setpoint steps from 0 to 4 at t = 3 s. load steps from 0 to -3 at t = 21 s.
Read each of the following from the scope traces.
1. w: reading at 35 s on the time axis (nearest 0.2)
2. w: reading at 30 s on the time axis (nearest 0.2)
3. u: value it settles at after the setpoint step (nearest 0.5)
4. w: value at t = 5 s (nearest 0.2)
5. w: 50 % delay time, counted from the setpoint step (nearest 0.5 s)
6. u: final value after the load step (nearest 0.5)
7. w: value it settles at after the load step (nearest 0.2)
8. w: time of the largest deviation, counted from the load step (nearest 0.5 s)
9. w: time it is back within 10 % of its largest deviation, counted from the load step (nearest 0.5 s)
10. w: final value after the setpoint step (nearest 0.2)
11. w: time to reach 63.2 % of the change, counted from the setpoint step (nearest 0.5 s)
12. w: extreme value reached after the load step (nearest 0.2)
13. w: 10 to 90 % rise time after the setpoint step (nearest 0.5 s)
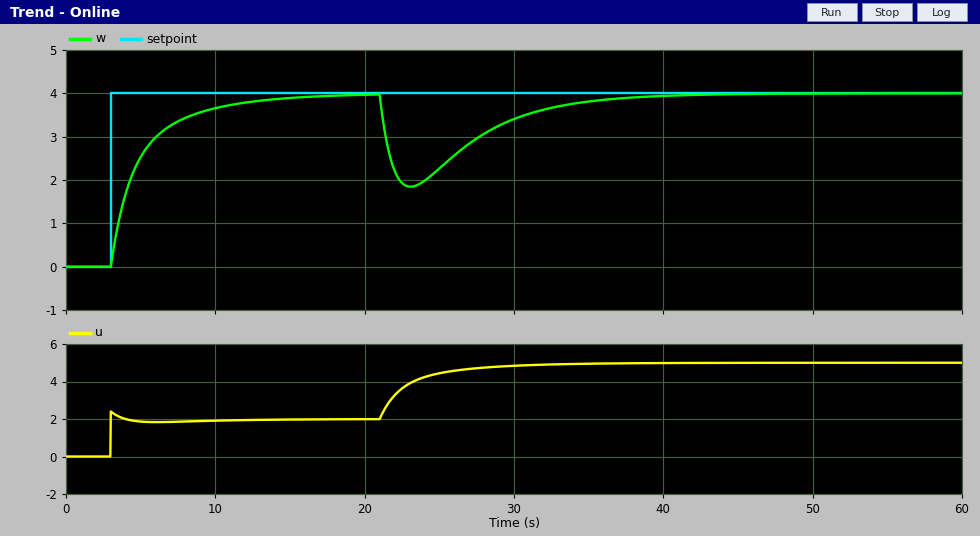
3.8
3.4
2.0
2.6
1.5 s
5.0
4.0
2.0 s
13.5 s
4.0
2.0 s
1.8
6.0 s
